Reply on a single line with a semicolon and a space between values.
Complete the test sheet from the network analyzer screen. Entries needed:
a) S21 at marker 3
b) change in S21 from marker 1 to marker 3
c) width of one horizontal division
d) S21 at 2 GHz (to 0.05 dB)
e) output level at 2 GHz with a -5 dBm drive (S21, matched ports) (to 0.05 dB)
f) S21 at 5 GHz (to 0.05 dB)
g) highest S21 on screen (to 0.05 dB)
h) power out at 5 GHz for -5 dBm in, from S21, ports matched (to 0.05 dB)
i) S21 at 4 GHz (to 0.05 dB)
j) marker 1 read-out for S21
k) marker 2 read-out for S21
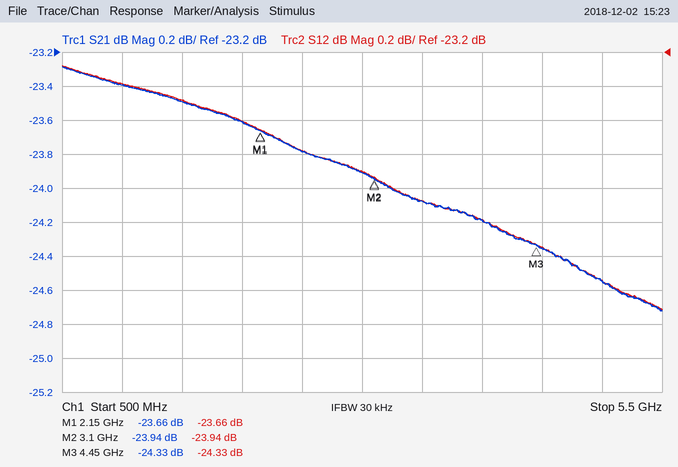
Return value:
-24.33 dB; -0.67 dB; 500 MHz; -23.60 dB; -28.60 dBm; -24.55 dB; -23.30 dB; -29.55 dBm; -24.20 dB; -23.66 dB; -23.94 dB
